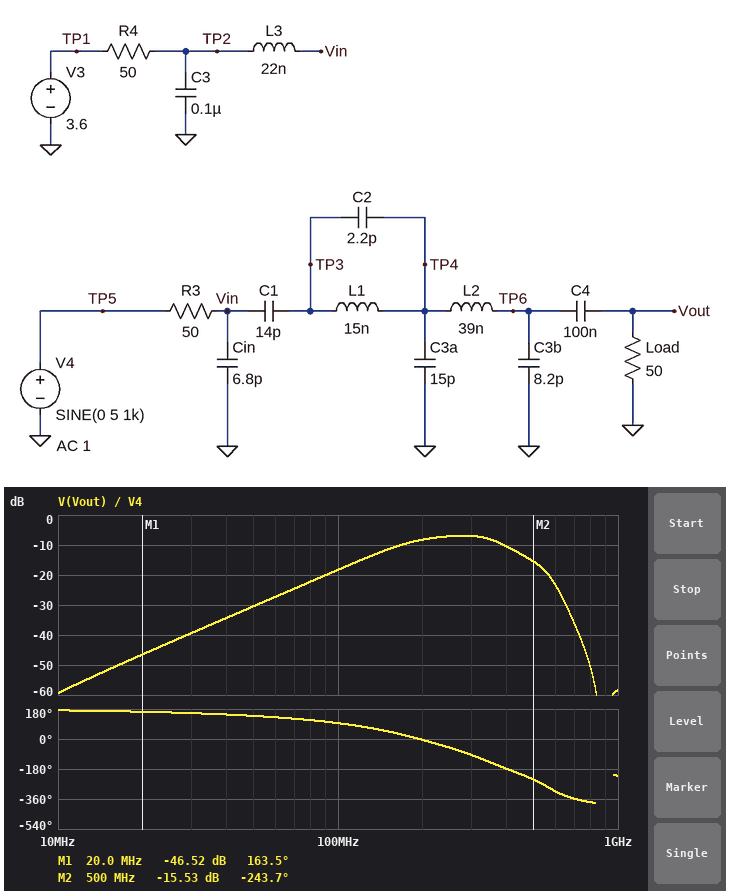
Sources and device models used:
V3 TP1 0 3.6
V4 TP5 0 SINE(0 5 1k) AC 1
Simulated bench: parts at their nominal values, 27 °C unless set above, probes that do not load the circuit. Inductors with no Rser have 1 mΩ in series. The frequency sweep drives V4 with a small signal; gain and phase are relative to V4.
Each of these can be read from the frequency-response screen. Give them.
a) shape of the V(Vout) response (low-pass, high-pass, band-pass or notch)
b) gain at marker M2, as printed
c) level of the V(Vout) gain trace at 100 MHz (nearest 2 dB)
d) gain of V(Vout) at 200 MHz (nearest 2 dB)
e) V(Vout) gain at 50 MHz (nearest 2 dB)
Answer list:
band-pass
-15.53 dB
-18 dB
-8 dB
-30 dB
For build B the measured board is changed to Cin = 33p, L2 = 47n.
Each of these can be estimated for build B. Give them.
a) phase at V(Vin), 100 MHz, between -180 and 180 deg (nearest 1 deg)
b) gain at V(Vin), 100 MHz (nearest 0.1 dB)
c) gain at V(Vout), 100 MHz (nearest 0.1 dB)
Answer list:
62 deg
-8.0 dB
-15.6 dB
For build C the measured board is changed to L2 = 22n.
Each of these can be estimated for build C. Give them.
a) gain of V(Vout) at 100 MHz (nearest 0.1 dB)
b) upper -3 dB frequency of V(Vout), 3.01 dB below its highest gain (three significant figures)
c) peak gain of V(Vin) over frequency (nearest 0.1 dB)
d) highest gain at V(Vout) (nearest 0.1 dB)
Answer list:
-19.2 dB
516 MHz
-0.2 dB
-6.1 dB
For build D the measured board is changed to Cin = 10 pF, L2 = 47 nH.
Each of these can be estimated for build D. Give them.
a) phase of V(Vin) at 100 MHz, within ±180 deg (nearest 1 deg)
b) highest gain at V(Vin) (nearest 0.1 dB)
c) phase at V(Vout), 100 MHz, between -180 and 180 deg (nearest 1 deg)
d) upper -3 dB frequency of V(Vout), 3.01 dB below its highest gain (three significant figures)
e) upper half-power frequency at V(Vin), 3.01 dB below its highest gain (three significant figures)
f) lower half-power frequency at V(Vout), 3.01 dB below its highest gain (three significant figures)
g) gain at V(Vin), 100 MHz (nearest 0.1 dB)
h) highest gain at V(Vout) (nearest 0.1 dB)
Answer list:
68 deg
-0.1 dB
91 deg
343 MHz
654 MHz
155 MHz
-10.0 dB
-7.5 dB
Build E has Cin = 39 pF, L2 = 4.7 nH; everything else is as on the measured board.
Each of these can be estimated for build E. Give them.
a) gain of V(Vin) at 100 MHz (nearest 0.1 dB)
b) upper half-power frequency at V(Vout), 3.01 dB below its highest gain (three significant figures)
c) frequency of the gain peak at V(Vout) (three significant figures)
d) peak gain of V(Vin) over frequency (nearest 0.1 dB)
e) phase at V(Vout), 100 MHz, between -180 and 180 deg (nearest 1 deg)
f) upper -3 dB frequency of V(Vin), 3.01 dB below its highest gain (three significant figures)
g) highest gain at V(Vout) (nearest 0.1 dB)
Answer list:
-7.3 dB
446 MHz
418 MHz
-1.3 dB
100 deg
188 MHz
-7.2 dB
